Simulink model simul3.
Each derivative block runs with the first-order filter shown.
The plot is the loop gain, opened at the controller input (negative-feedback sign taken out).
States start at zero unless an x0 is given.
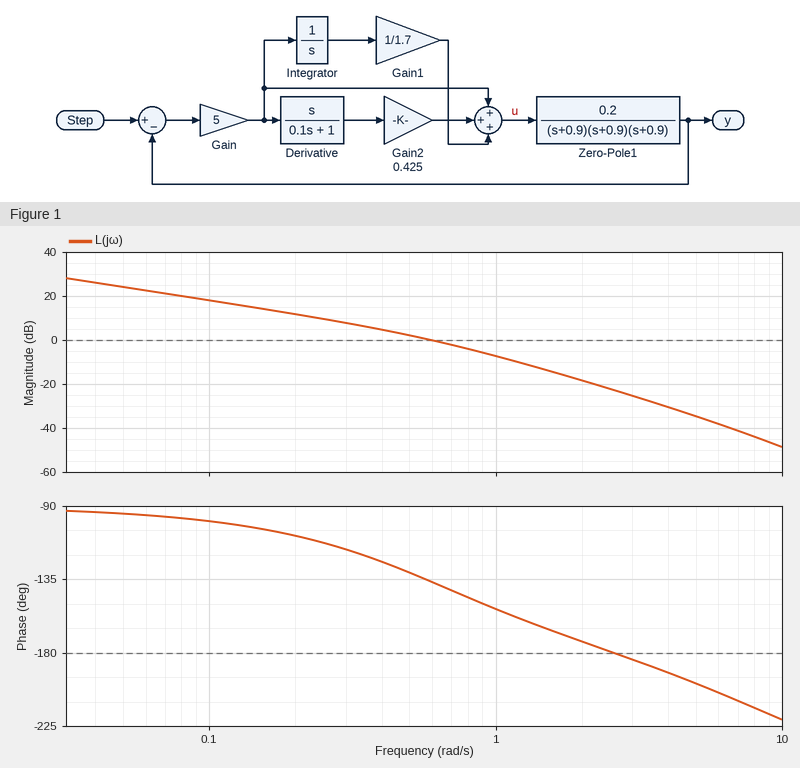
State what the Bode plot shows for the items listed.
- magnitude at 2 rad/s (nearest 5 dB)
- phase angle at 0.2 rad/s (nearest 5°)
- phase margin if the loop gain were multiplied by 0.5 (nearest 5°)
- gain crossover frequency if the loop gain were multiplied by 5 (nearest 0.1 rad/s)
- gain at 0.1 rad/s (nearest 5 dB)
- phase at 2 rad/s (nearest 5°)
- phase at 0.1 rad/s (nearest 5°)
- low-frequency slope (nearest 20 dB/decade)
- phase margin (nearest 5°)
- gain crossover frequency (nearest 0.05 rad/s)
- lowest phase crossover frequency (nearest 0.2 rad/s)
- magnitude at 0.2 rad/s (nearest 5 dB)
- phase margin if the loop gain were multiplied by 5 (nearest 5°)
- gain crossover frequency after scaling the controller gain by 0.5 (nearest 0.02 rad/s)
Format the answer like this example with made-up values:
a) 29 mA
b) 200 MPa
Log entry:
a) -20 dB
b) -110°
c) 60°
d) 1.5 rad/s
e) 20 dB
f) -175°
g) -100°
h) -20 dB/decade
i) 45°
j) 0.60 rad/s
k) 2.6 rad/s
l) 10 dB
m) 15°
n) 0.36 rad/s
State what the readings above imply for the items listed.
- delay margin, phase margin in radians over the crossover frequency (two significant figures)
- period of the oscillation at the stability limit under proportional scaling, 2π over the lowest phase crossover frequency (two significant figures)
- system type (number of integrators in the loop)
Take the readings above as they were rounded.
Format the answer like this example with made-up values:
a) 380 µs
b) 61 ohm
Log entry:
a) 1.3 s
b) 2.4 s
c) 1
